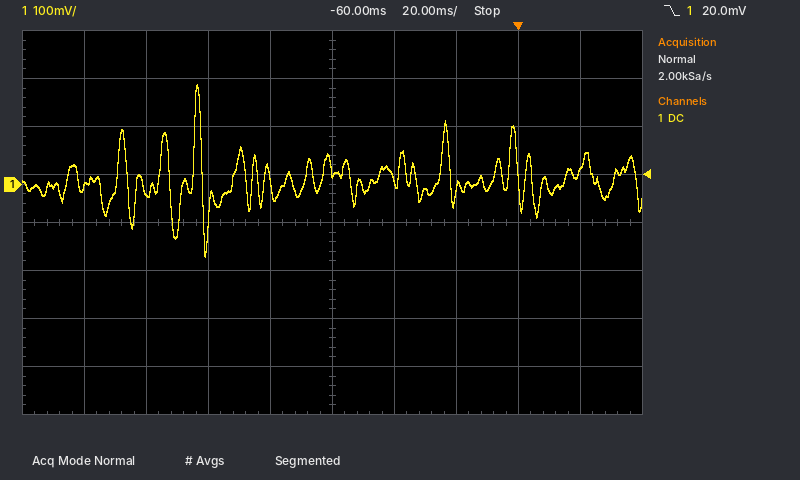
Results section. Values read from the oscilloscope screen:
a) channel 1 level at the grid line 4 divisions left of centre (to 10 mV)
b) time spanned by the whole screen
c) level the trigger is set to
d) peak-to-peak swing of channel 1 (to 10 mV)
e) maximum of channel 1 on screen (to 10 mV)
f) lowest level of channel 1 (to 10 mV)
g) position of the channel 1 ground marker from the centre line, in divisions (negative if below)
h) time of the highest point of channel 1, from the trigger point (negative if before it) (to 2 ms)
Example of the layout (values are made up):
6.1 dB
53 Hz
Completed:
-10 mV
200 ms
20.0 mV
360 mV
210 mV
-150 mV
+0.8 div
-104 ms
